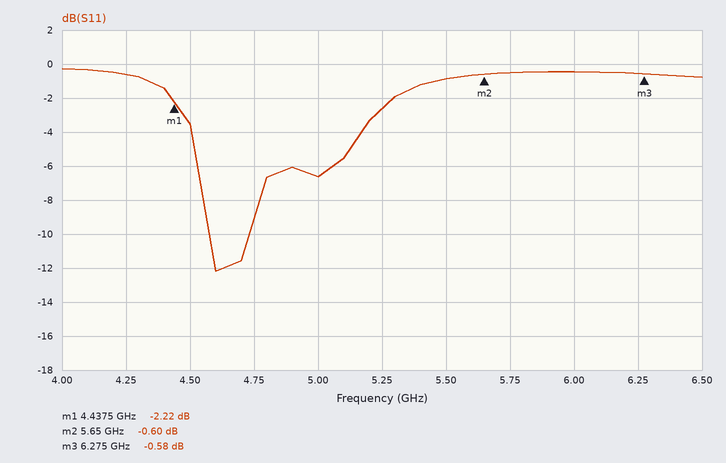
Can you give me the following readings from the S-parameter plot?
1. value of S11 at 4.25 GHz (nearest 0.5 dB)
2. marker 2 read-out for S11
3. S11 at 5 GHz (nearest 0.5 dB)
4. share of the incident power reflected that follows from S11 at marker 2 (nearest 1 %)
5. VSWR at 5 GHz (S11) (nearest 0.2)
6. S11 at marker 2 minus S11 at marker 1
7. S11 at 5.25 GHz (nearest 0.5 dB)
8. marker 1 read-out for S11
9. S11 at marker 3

-0.5 dB
-0.60 dB
-6.5 dB
87 %
2.8
1.62 dB
-2.5 dB
-2.22 dB
-0.58 dB
